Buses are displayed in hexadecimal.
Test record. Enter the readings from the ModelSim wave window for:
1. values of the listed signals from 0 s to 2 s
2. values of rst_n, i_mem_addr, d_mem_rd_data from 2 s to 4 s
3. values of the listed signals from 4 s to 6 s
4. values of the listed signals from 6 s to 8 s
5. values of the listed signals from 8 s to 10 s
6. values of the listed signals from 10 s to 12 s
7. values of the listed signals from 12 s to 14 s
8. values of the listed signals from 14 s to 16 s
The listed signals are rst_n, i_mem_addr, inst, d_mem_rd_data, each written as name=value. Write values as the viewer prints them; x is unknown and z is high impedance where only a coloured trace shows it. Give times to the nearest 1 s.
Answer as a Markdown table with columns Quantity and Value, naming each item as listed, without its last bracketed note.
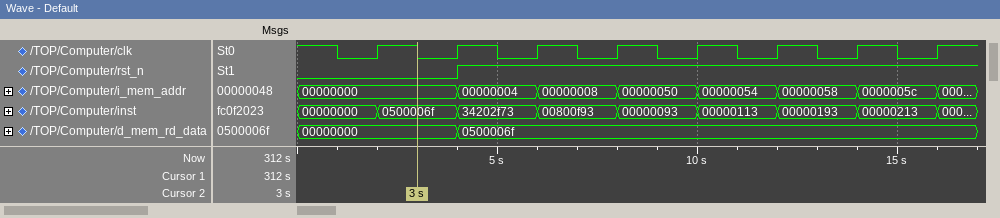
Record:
| Quantity | Value |
|---|---|
| values of the listed signals from 0 s to 2 s | rst_n=0, i_mem_addr=00000000, inst=00000000, d_mem_rd_data=00000000 |
| values of rst_n, i_mem_addr, d_mem_rd_data from 2 s to 4 s | rst_n=0, i_mem_addr=00000000, d_mem_rd_data=00000000 |
| values of the listed signals from 4 s to 6 s | rst_n=1, i_mem_addr=00000004, inst=34202f73, d_mem_rd_data=0500006f |
| values of the listed signals from 6 s to 8 s | rst_n=1, i_mem_addr=00000008, inst=00800f93, d_mem_rd_data=0500006f |
| values of the listed signals from 8 s to 10 s | rst_n=1, i_mem_addr=00000050, inst=00000093, d_mem_rd_data=0500006f |
| values of the listed signals from 10 s to 12 s | rst_n=1, i_mem_addr=00000054, inst=00000113, d_mem_rd_data=0500006f |
| values of the listed signals from 12 s to 14 s | rst_n=1, i_mem_addr=00000058, inst=00000193, d_mem_rd_data=0500006f |
| values of the listed signals from 14 s to 16 s | rst_n=1, i_mem_addr=0000005c, inst=00000213, d_mem_rd_data=0500006f |
